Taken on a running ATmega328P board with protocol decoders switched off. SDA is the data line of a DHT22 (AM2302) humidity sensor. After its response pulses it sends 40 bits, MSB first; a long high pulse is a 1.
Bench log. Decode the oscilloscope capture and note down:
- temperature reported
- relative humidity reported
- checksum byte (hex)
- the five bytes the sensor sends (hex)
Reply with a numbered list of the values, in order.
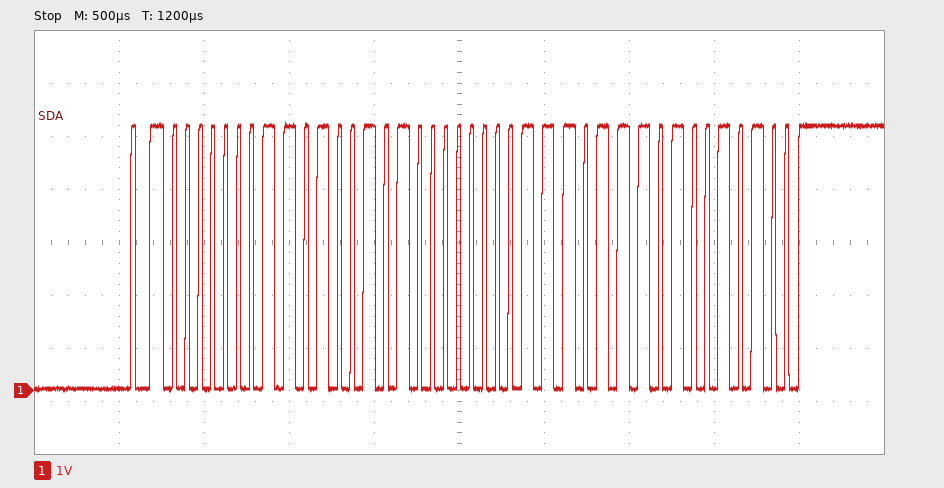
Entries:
1. 23.8 °C
2. 42.1 %
3. 0x94
4. 01 A5 00 EE 94
